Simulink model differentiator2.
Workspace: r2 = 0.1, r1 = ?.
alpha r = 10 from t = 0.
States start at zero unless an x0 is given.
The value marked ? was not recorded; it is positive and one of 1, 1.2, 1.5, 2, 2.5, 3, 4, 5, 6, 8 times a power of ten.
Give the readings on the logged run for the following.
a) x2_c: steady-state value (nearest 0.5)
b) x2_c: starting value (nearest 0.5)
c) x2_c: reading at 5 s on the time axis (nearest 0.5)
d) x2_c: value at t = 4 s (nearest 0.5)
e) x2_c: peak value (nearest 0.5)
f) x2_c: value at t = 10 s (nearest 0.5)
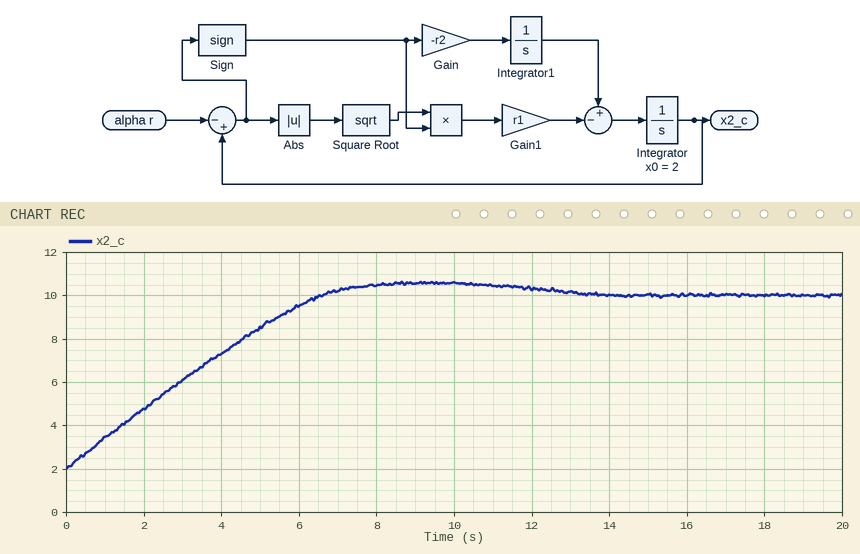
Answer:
10.0
2.0
8.5
7.5
10.5
10.5
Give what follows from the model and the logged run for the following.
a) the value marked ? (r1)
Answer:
0.5
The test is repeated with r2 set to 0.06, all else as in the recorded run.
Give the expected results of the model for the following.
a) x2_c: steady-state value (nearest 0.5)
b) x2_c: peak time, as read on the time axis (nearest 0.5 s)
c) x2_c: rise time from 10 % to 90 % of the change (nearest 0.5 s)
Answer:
10.0
10.0 s
5.5 s
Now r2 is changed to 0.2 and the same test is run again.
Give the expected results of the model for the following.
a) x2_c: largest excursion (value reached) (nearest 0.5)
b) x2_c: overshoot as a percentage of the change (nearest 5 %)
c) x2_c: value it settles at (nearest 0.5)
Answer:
11.0
15 %
10.0
